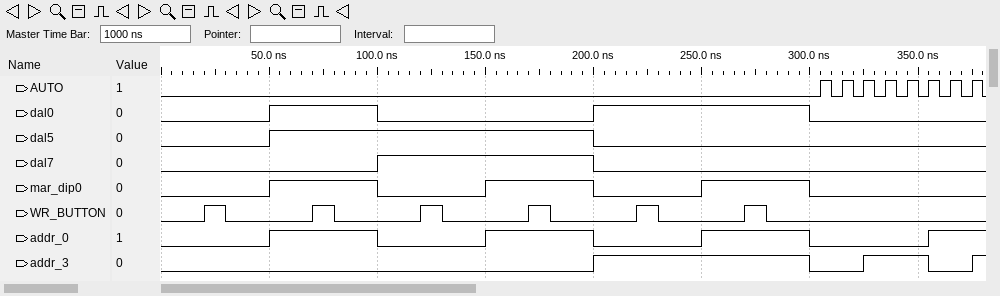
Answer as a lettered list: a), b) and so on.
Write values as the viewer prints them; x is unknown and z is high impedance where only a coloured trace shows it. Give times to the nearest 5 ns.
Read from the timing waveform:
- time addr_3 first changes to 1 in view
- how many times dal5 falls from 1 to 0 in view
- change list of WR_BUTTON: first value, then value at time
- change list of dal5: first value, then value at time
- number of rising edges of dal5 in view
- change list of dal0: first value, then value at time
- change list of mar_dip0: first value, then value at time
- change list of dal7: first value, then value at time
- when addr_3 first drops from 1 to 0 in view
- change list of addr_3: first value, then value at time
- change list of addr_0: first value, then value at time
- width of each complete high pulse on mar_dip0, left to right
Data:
a) 200 ns
b) 1
c) 0, 1 at 20 ns, 0 at 30 ns, 1 at 70 ns, 0 at 80 ns, 1 at 120 ns, 0 at 130 ns, 1 at 170 ns, 0 at 180 ns, 1 at 220 ns, 0 at 230 ns, 1 at 270 ns, 0 at 280 ns
d) 0, 1 at 50 ns, 0 at 200 ns
e) 1
f) 0, 1 at 50 ns, 0 at 100 ns, 1 at 200 ns, 0 at 300 ns
g) 0, 1 at 50 ns, 0 at 100 ns, 1 at 150 ns, 0 at 200 ns, 1 at 250 ns, 0 at 300 ns
h) 0, 1 at 100 ns, 0 at 200 ns
i) 300 ns
j) 0, 1 at 200 ns, 0 at 300 ns, 1 at 325 ns, 0 at 355 ns, 1 at 375 ns
k) 0, 1 at 50 ns, 0 at 100 ns, 1 at 150 ns, 0 at 200 ns, 1 at 250 ns, 0 at 300 ns, 1 at 355 ns
l) 50 ns, 50 ns, 50 ns
